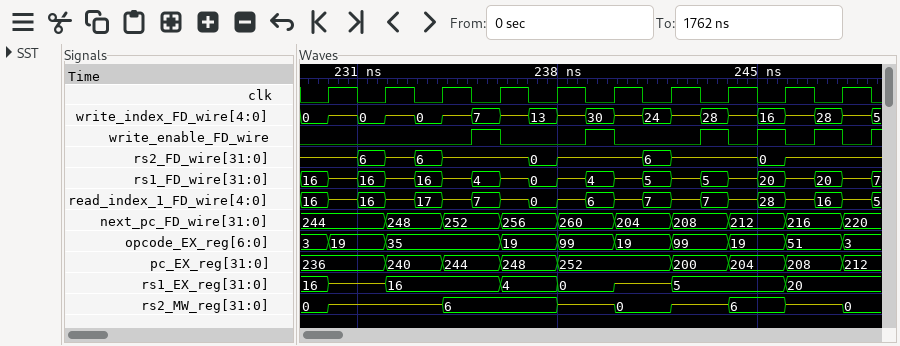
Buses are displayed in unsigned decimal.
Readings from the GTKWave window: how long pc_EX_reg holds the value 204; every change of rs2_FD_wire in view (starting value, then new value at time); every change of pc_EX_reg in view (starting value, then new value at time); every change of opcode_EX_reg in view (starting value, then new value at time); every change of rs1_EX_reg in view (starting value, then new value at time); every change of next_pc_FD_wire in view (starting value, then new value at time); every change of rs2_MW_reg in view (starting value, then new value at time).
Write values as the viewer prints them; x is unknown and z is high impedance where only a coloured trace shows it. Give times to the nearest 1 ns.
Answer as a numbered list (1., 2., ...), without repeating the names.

1. 2 ns
2. z, 6 at 231 ns, z at 232 ns, 6 at 233 ns, z at 234 ns, 0 at 237 ns, z at 238 ns, 6 at 241 ns, z at 242 ns, 0 at 245 ns, z at 246 ns
3. 236, 240 at 232 ns, 244 at 234 ns, 248 at 236 ns, 252 at 238 ns, 200 at 242 ns, 204 at 244 ns, 208 at 246 ns, 212 at 248 ns
4. 3, 19 at 230 ns, 35 at 232 ns, 19 at 236 ns, 99 at 238 ns, 19 at 240 ns, 99 at 242 ns, 19 at 244 ns, 51 at 246 ns, 3 at 248 ns
5. 16, z at 230 ns, 16 at 232 ns, 4 at 236 ns, 0 at 238 ns, z at 240 ns, 5 at 242 ns, 20 at 246 ns
6. 244, 248 at 232 ns, 252 at 234 ns, 256 at 236 ns, 260 at 238 ns, 204 at 240 ns, 208 at 242 ns, 212 at 244 ns, 216 at 246 ns, 220 at 248 ns
7. 0, z at 230 ns, 6 at 234 ns, z at 238 ns, 0 at 240 ns, z at 242 ns, 6 at 244 ns, z at 246 ns, 0 at 248 ns
